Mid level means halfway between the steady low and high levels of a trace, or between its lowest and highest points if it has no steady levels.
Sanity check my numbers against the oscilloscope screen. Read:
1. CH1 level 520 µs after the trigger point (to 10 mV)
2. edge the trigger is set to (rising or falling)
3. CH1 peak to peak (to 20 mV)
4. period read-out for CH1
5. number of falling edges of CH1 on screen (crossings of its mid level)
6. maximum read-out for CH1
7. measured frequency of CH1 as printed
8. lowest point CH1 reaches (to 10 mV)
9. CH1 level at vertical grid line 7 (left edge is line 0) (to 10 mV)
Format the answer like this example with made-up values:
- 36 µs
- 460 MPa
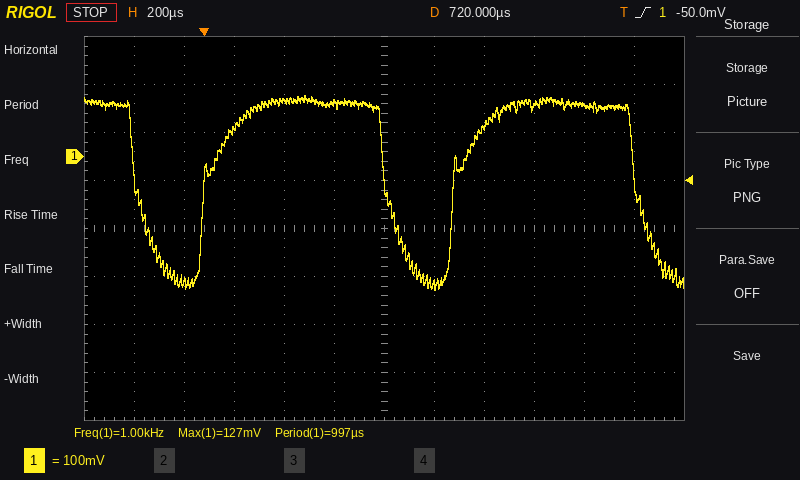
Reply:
- 110 mV
- rising
- 400 mV
- 997 µs
- 3
- 127 mV
- 1.00 kHz
- -280 mV
- -270 mV
